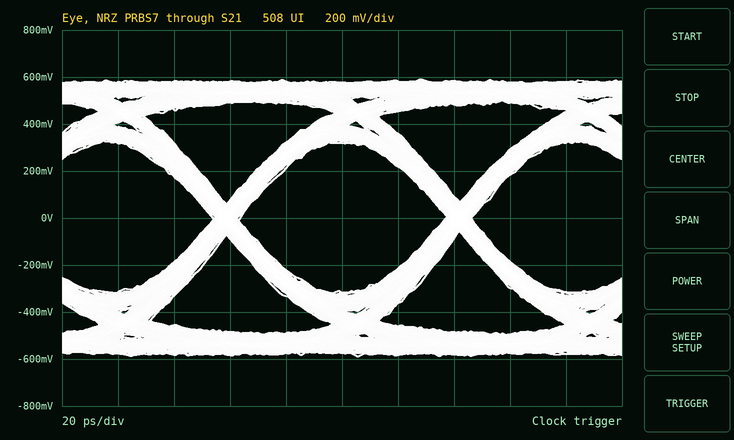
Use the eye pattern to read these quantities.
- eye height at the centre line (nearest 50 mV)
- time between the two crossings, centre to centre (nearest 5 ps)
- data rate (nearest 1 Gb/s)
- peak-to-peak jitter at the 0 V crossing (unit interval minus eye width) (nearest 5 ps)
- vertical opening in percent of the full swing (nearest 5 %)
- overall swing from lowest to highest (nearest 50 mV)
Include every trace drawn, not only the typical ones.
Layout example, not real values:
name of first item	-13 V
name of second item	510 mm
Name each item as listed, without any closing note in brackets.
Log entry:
eye height at the centre line	650 mV
time between the two crossings, centre to centre	85 ps
data rate	12 Gb/s
peak-to-peak jitter at the 0 V crossing (unit interval minus eye width)	10 ps
vertical opening in percent of the full swing	55 %
overall swing from lowest to highest	1.20 V
